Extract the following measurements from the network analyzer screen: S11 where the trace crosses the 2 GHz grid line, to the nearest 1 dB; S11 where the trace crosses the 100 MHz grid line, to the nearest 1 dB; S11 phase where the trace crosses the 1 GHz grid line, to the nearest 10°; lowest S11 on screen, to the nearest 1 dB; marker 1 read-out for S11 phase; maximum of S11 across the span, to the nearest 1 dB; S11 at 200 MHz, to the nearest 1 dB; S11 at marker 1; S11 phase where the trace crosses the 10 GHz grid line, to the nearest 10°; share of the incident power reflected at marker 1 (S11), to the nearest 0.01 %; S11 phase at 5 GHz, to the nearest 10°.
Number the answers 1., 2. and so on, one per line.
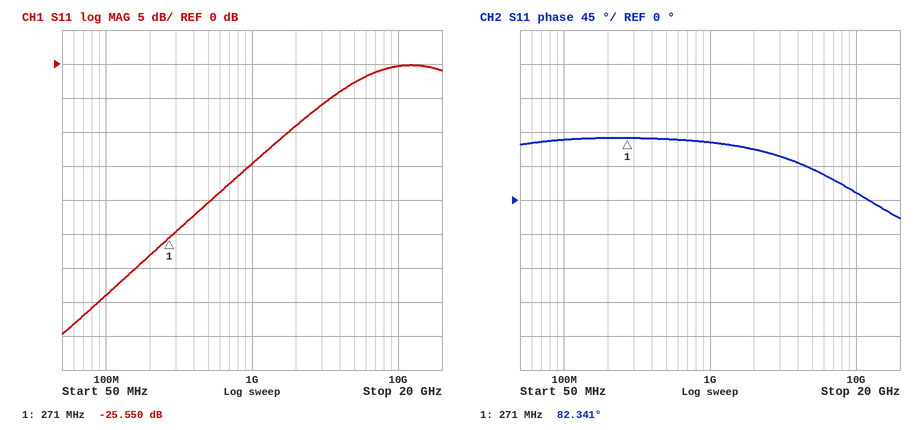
1. -9 dB
2. -34 dB
3. 80°
4. -40 dB
5. 82.341°
6. 0 dB
7. -28 dB
8. -25.550 dB
9. 10°
10. 0.28 %
11. 40°
